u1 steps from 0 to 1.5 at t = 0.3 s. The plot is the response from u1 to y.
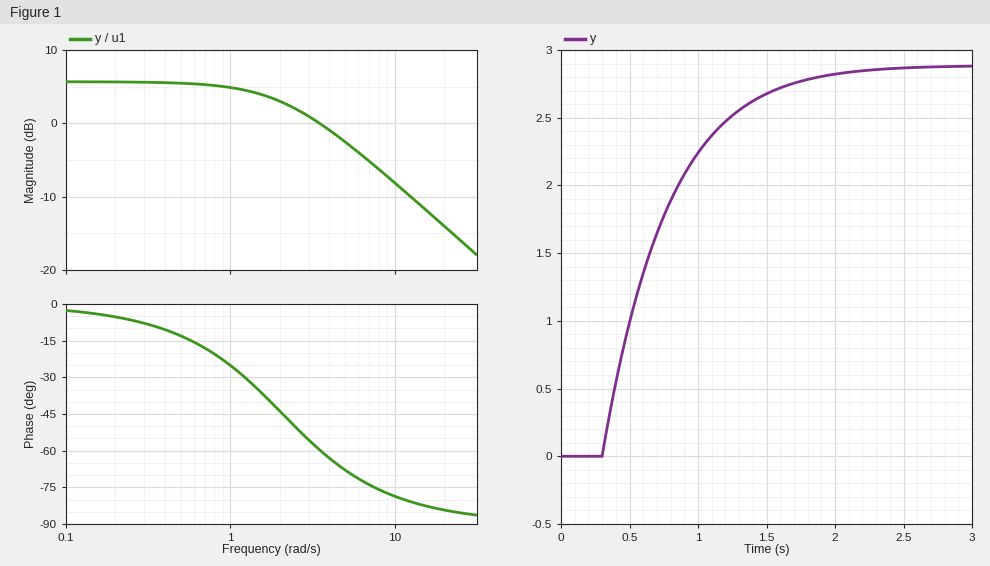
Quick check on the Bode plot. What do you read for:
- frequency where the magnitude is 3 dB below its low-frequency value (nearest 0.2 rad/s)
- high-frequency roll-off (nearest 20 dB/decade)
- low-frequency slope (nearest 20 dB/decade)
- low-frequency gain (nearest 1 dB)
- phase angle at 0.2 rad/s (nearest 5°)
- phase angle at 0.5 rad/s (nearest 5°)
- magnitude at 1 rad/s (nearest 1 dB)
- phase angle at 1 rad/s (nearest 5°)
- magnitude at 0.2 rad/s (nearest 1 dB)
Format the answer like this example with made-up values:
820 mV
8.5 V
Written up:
2.2 rad/s
-20 dB/decade
0 dB/decade
6 dB
-5°
-15°
5 dB
-25°
6 dB
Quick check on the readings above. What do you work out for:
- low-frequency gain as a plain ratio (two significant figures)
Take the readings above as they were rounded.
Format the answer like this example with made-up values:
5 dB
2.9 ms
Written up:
2.0
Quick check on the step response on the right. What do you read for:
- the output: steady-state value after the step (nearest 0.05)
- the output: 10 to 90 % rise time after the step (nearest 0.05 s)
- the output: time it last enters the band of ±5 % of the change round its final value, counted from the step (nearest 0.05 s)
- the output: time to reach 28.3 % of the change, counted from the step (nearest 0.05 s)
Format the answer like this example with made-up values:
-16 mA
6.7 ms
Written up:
2.90
1.00 s
1.35 s
0.15 s
